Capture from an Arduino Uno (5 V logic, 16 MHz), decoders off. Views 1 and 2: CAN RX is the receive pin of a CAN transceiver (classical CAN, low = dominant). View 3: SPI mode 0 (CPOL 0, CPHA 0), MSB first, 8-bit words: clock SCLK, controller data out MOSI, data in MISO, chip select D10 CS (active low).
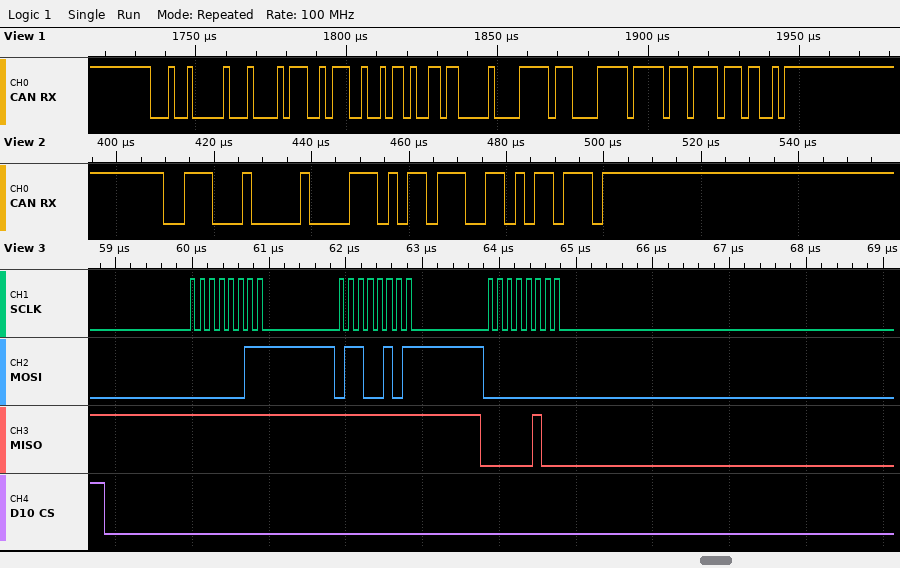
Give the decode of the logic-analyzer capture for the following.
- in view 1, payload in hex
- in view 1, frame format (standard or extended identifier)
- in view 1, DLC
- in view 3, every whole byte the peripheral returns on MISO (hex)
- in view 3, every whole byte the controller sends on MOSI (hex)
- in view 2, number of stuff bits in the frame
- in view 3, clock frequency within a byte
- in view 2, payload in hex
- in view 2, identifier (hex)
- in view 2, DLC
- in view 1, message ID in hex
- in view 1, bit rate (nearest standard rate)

5C B9 2D 36 00 FF 0F FF
standard
8
FF FF 04
03 65 00
1
8 MHz
D6
0x388
1
0x120
500 kbit/s
